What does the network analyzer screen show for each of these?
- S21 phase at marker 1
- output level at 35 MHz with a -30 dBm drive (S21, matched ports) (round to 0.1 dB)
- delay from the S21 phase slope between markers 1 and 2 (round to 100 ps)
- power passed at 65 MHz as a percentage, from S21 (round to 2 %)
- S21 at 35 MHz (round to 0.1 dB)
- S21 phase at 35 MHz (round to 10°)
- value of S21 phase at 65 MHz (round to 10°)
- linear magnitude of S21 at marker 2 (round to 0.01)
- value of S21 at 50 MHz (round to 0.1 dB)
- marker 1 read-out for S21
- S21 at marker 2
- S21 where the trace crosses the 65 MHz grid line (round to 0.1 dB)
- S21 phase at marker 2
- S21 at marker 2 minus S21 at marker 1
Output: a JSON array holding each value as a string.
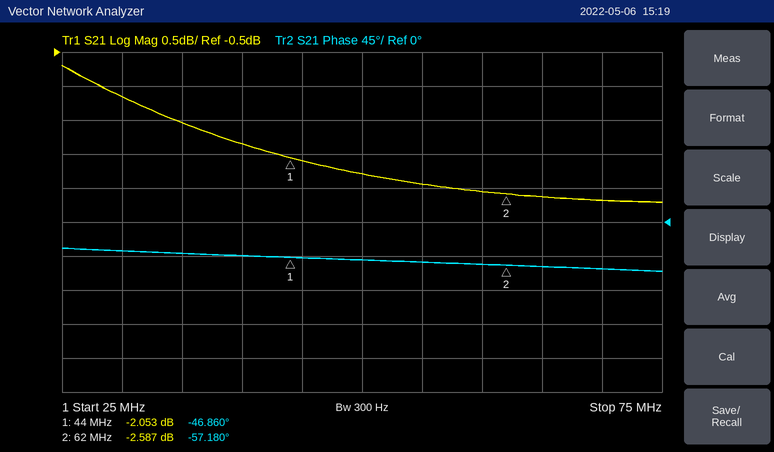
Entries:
["-46.860°", "-31.5 dBm", "1.6 ns", "54 %", "-1.5 dB", "-40°", "-60°", "0.74", "-2.3 dB", "-2.053 dB", "-2.587 dB", "-2.6 dB", "-57.180°", "-0.534 dB"]
